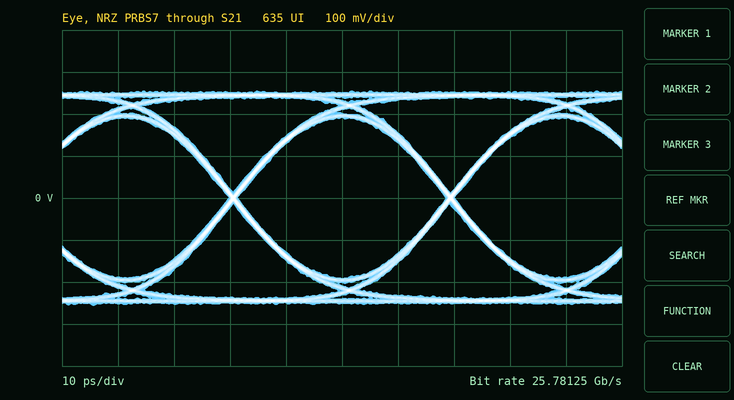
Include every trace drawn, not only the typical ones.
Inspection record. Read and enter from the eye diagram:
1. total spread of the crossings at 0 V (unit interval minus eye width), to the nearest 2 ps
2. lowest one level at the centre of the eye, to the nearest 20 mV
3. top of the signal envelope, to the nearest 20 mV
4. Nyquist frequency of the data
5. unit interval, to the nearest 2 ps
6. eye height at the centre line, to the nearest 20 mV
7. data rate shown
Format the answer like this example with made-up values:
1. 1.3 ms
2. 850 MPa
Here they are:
1. 2 ps
2. 200 mV
3. 260 mV
4. 12.89062 GHz
5. 38 ps
6. 380 mV
7. 25.78125 Gb/s
